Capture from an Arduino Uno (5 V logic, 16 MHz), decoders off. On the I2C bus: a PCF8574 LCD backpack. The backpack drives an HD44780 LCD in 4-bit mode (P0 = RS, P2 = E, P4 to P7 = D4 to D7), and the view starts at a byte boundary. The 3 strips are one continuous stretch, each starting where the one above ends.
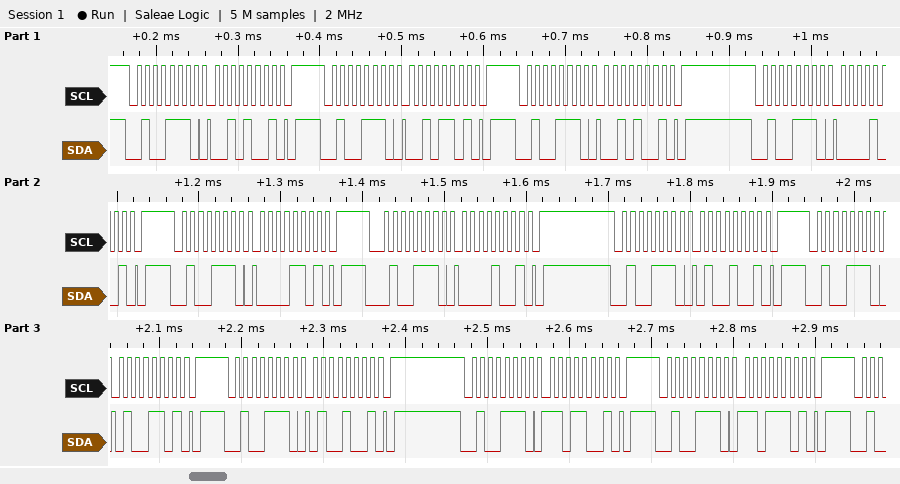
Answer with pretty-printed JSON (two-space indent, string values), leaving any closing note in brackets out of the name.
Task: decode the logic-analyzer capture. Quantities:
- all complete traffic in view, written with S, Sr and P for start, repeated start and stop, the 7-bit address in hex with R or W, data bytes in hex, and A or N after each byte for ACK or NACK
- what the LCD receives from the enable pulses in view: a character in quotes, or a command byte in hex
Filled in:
{
  "all complete traffic in view, written with S, Sr and P for start, repeated start and stop, the 7-bit address in hex with R or W, data bytes in hex, and A or N after each byte for ACK or NACK": "S 27W A 29 A P S 27W A 2D A P S 27W A 29 A P S 27W A 09 A P S 27W A 0D A P S 27W A 09 A P S 27W A 49 A P S 27W A 4D A P S 27W A 49 A P S 27W A D9 A P S 27W A DD A P",
  "what the LCD receives from the enable pulses in view: a character in quotes, or a command byte in hex": "' '"
}
